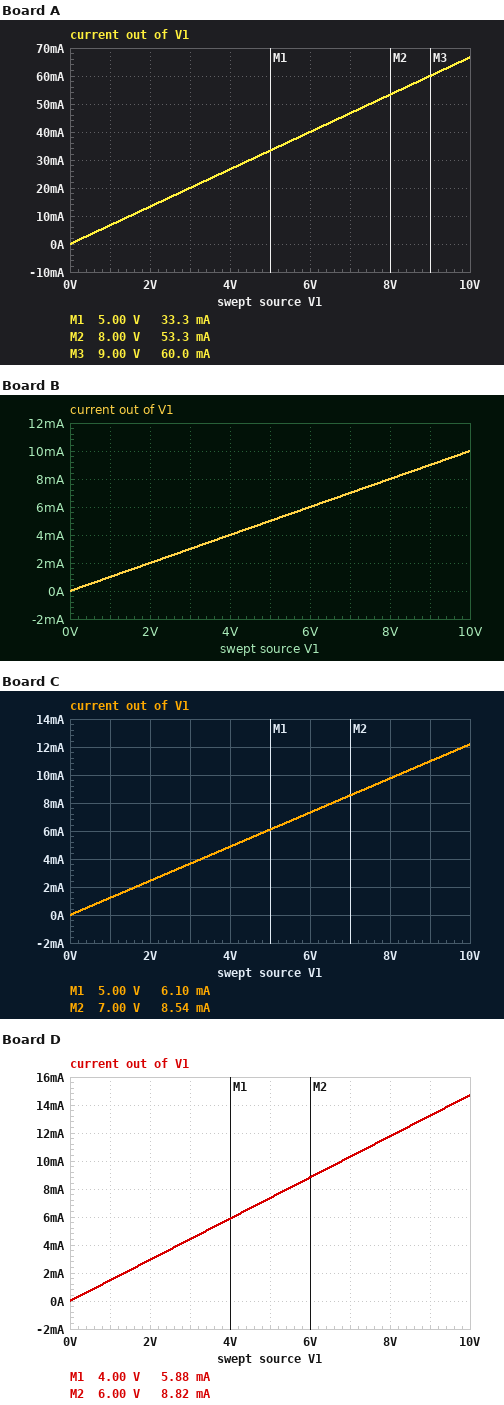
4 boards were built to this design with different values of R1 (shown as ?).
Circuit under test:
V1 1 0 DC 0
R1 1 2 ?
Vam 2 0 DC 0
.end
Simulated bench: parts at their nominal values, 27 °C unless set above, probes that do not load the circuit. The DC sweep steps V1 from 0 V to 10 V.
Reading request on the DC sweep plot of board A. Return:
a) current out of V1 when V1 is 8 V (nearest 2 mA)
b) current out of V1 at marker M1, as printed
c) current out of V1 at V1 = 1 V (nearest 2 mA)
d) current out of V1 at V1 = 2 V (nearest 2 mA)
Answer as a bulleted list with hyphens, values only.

- 54 mA
- 33.3 mA
- 6 mA
- 14 mA
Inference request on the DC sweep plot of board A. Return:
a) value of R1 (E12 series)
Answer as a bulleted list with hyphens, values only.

- 150 Ω
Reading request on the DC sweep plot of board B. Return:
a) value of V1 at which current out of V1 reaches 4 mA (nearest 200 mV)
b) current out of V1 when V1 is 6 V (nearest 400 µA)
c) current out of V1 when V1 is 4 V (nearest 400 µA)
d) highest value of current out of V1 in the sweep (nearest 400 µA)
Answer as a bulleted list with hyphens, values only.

- 4.0 V
- 6.0 mA
- 4.0 mA
- 10.0 mA
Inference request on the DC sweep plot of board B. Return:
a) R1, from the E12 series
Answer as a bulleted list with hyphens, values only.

- 1 kΩ
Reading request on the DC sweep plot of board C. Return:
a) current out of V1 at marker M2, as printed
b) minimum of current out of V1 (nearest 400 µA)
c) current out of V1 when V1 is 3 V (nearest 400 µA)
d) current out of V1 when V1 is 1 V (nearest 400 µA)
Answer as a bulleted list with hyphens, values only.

- 8.54 mA
- 0 A
- 3.6 mA
- 1.2 mA
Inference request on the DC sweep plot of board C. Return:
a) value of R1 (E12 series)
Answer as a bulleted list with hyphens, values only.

- 820 Ω
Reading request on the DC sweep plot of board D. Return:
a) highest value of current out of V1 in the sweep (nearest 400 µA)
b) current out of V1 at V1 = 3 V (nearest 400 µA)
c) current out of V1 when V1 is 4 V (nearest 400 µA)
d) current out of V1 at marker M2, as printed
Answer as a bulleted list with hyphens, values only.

- 14.8 mA
- 4.4 mA
- 6.0 mA
- 8.82 mA
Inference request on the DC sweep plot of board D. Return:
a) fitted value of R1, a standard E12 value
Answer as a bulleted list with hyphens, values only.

- 680 Ω
